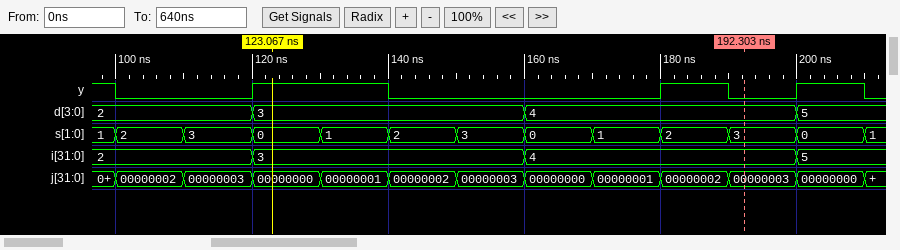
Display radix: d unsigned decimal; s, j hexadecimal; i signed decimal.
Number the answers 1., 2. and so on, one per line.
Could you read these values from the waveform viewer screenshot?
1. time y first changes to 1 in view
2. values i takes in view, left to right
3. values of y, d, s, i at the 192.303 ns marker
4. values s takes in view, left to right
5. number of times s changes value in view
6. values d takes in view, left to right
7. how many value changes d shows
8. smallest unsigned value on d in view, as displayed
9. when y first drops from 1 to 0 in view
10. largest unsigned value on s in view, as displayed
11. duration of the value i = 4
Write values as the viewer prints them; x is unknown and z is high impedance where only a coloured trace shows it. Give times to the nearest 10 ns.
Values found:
1. 120 ns
2. 2, 3, 4, 5
3. y=0, d=4, s=3, i=4
4. 1, 2, 3, 0, 1, 2, 3, 0, 1, 2, 3, 0, 1
5. 12
6. 2, 3, 4, 5
7. 3
8. 2
9. 100 ns
10. 3
11. 40 ns
